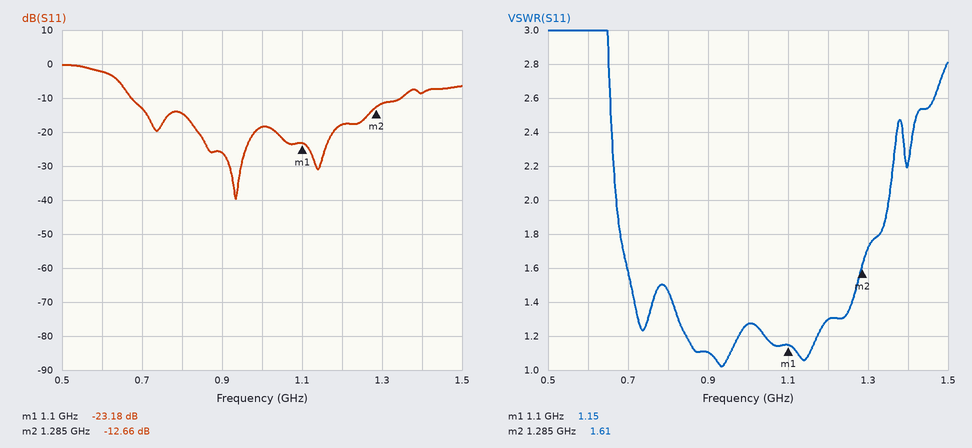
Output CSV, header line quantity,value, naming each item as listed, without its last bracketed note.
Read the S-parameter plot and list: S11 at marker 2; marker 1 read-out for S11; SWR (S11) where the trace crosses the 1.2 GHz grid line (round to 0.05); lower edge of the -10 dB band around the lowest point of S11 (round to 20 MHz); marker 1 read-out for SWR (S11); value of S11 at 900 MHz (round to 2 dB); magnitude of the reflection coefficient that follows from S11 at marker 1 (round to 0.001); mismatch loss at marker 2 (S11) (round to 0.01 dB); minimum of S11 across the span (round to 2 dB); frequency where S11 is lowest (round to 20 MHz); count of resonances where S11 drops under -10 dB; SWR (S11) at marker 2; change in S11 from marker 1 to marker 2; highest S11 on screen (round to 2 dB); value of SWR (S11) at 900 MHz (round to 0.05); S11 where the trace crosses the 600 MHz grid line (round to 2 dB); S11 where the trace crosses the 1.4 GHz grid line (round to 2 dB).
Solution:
quantity,value
S11 at marker 2,-12.66 dB
marker 1 read-out for S11,-23.18 dB
SWR (S11) where the trace crosses the 1.2 GHz grid line,1.30
lower edge of the -10 dB band around the lowest point of S11,680 MHz
marker 1 read-out for SWR,1.15
value of S11 at 900 MHz,-26 dB
magnitude of the reflection coefficient that follows from S11 at marker 1,0.069
mismatch loss at marker 2 (S11),0.24 dB
minimum of S11 across the span,-40 dB
frequency where S11 is lowest,940 MHz
count of resonances where S11 drops under -10 dB,3
SWR (S11) at marker 2,1.61
change in S11 from marker 1 to marker 2,10.52 dB
highest S11 on screen,0 dB
value of SWR (S11) at 900 MHz,1.10
S11 where the trace crosses the 600 MHz grid line,-2 dB
S11 where the trace crosses the 1.4 GHz grid line,-8 dB
